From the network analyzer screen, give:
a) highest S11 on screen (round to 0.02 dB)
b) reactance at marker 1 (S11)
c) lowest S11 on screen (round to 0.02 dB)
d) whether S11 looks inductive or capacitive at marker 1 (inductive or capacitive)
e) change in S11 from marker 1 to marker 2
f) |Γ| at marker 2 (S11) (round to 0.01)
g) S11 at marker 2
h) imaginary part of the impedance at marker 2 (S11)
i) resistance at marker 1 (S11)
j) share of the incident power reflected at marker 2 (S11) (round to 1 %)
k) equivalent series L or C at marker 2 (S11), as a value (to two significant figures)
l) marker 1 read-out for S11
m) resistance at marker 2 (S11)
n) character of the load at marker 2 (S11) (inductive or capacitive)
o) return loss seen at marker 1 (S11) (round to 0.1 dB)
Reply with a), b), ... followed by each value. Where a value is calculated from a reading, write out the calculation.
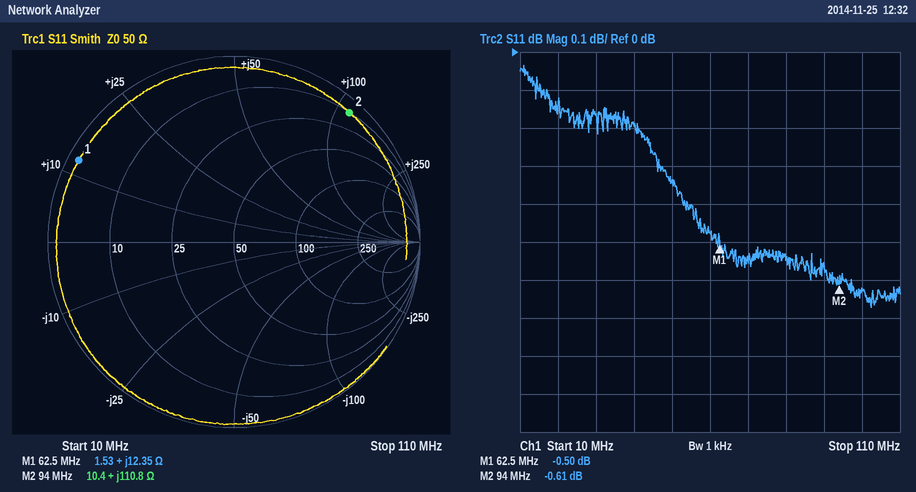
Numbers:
a) -0.04 dB
b) +12.35 Ω
c) -0.68 dB
d) inductive
e) -0.61 − (-0.5) = -0.11 dB
f) 0.93
g) -0.61 dB
h) +110.8 Ω
i) 1.53 Ω
j) 10^(-0.61/10) ≈ 87 %
k) L = 110.8 Ω/(2π × 94 MHz) ≈ 188 nH, so 190 nH to two significant figures
l) -0.50 dB
m) 10.4 Ω
n) inductive
o) 0.5 dB
